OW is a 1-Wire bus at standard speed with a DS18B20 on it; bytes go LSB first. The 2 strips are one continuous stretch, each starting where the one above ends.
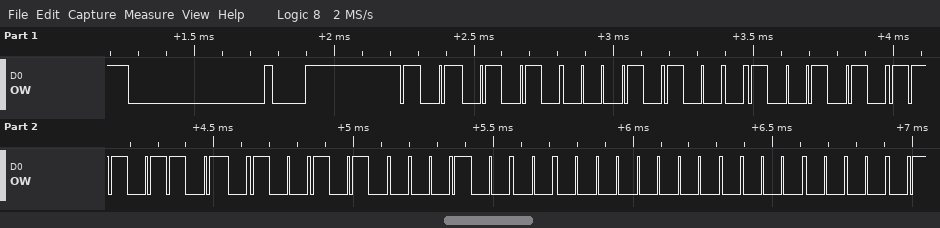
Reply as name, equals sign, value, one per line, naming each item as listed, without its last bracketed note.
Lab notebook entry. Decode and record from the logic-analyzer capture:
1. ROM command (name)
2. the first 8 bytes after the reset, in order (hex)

ROM command = Match ROM
the first 8 bytes after the reset, in order = 55 28 52 B7 52 08 00 00
